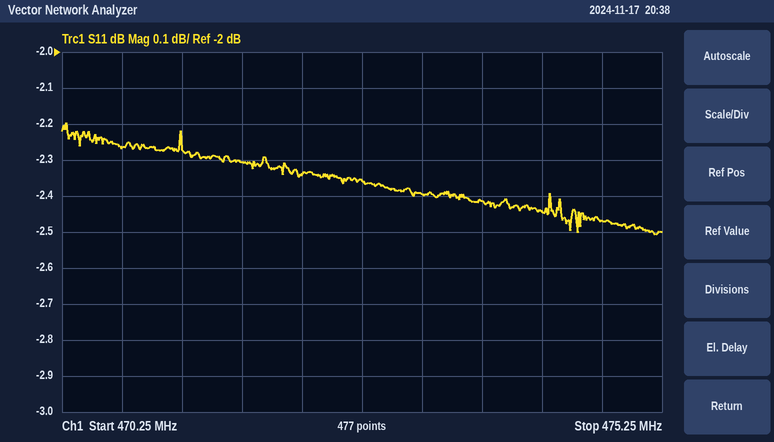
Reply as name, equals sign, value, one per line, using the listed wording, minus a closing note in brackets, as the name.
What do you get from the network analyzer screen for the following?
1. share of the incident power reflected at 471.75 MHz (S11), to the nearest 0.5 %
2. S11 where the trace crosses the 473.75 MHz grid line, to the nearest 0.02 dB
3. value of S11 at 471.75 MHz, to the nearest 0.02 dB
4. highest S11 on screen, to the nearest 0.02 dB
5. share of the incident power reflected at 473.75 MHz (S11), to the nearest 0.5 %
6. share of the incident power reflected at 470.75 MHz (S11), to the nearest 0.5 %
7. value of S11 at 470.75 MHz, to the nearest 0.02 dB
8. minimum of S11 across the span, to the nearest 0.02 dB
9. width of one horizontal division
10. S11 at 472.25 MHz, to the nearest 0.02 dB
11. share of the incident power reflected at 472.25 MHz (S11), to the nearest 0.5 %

share of the incident power reflected at 471.75 MHz (S11), to the nearest 0.5 % = 59.0 %
S11 where the trace crosses the 473.75 MHz grid line, to the nearest 0.02 dB = -2.42 dB
value of S11 at 471.75 MHz, to the nearest 0.02 dB = -2.30 dB
highest S11 on screen, to the nearest 0.02 dB = -2.20 dB
share of the incident power reflected at 473.75 MHz (S11), to the nearest 0.5 % = 57.5 %
share of the incident power reflected at 470.75 MHz (S11), to the nearest 0.5 % = 59.5 %
value of S11 at 470.75 MHz, to the nearest 0.02 dB = -2.26 dB
minimum of S11 across the span, to the nearest 0.02 dB = -2.50 dB
width of one horizontal division = 500 kHz
S11 at 472.25 MHz, to the nearest 0.02 dB = -2.34 dB
share of the incident power reflected at 472.25 MHz (S11), to the nearest 0.5 % = 58.5 %
